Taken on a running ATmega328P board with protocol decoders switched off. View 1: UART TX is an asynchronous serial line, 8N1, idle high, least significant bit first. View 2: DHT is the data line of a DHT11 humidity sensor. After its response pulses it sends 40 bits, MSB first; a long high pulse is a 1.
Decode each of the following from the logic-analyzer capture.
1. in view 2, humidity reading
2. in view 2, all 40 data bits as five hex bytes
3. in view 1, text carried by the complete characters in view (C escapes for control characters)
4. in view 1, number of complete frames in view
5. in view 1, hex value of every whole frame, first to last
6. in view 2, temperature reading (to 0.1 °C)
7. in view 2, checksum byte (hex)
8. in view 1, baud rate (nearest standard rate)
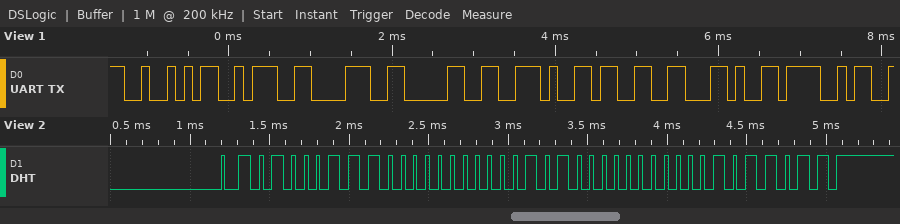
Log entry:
71 %
47 00 14 00 5B
"R:80.3,O"
8
52 3A 38 30 2E 33 2C 4F
20.0 °C
0x5B
9600 baud
